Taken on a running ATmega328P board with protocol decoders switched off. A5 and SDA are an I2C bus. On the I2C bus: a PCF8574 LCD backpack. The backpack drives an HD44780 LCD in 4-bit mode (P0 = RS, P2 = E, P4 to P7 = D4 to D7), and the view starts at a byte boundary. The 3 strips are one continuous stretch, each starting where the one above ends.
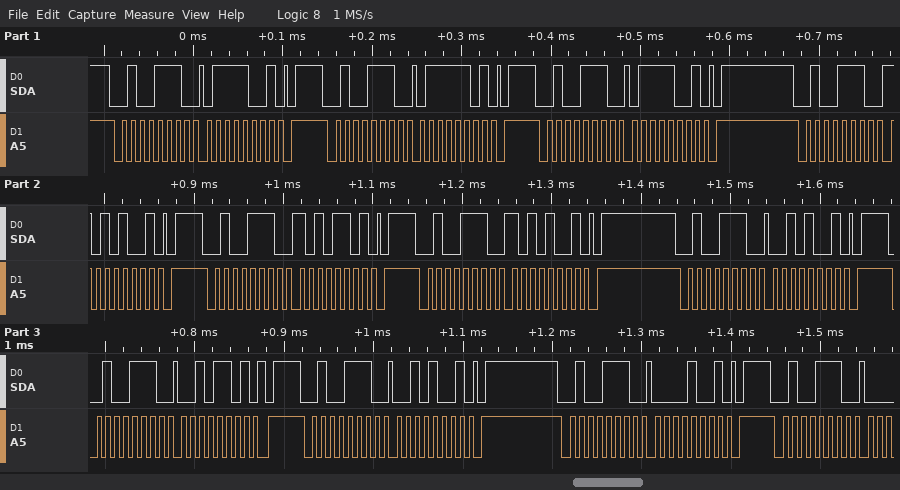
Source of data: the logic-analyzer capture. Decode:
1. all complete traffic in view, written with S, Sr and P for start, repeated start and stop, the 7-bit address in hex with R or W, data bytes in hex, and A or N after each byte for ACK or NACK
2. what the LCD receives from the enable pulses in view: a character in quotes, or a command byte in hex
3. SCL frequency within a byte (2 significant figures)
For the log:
S 27W A 79 A P S 27W A 7D A P S 27W A 79 A P S 27W A A9 A P S 27W A AD A P S 27W A A9 A P S 27W A 29 A P S 27W A 2D A P S 27W A 29 A P S 27W A 09 A P S 27W A
'z'
100 kHz
